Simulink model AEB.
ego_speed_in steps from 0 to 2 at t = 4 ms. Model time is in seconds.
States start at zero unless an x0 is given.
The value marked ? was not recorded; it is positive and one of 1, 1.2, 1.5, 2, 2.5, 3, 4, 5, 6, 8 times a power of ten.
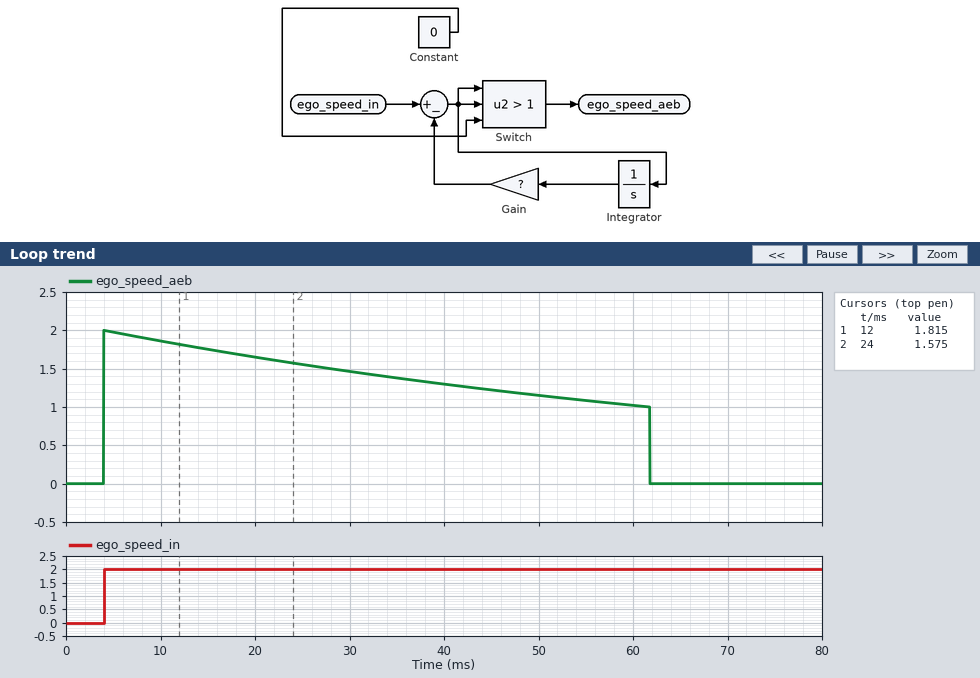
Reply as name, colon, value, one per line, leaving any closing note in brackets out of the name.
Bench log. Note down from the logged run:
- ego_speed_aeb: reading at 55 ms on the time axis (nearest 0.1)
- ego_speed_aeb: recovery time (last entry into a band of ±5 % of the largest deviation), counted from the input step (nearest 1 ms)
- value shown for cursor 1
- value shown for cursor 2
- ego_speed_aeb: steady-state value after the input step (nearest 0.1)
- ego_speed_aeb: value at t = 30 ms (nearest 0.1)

ego_speed_aeb: reading at 55 ms on the time axis: 1.1
ego_speed_aeb: recovery time (last entry into a band of ±5 % of the largest deviation), counted from the input step: 58 ms
value shown for cursor 1: 1.815
value shown for cursor 2: 1.575
ego_speed_aeb: steady-state value after the input step: 0.0
ego_speed_aeb: value at t = 30 ms: 1.5
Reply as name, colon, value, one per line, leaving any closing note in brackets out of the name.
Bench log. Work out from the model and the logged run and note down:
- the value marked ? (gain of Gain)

the value marked ?: 12
